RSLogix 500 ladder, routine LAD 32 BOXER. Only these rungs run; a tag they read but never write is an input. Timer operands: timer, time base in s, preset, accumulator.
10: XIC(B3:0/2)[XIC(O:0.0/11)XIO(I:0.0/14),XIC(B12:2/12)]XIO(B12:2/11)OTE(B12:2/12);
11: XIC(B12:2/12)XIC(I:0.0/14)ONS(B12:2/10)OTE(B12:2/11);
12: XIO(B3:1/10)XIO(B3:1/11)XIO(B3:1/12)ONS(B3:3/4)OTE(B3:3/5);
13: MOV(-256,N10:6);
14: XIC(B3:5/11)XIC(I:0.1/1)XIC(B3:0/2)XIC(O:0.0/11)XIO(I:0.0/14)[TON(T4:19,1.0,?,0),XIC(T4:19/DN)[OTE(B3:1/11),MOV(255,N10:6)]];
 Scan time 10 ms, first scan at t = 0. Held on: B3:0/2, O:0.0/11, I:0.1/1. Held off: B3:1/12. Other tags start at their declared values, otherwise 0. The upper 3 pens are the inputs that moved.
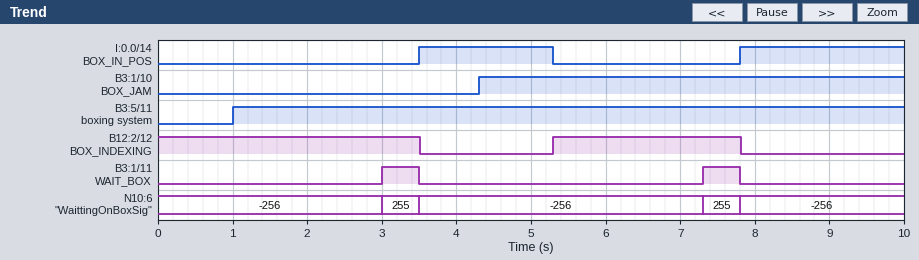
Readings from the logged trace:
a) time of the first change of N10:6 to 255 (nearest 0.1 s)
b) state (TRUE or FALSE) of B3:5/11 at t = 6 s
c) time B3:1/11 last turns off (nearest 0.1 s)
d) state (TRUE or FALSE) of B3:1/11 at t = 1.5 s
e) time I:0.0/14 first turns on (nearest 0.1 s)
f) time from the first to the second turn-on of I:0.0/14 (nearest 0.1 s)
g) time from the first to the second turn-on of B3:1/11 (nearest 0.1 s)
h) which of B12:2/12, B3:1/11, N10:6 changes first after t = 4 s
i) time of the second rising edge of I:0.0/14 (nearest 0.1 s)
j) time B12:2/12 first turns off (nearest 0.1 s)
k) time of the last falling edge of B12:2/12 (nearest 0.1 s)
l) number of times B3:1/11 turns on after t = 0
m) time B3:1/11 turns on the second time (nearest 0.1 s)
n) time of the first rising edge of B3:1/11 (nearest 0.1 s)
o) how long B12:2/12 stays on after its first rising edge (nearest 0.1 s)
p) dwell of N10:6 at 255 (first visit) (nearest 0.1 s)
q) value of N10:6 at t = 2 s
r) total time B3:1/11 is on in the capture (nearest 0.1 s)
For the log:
3.0 s
TRUE
7.8 s
FALSE
3.5 s
4.3 s
4.3 s
B12:2/12
7.8 s
3.5 s
7.8 s
2
7.3 s
3.0 s
2.5 s
0.5 s
-256
1.0 s
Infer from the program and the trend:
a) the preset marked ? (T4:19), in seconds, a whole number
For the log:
2 s
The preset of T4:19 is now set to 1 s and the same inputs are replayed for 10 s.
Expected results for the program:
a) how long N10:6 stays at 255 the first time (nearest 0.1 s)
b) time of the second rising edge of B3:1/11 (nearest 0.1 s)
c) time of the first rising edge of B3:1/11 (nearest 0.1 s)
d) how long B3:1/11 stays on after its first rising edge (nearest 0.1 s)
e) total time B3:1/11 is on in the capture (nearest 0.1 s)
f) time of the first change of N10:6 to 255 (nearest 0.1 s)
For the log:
1.5 s
6.3 s
2.0 s
1.5 s
3.0 s
2.0 s
